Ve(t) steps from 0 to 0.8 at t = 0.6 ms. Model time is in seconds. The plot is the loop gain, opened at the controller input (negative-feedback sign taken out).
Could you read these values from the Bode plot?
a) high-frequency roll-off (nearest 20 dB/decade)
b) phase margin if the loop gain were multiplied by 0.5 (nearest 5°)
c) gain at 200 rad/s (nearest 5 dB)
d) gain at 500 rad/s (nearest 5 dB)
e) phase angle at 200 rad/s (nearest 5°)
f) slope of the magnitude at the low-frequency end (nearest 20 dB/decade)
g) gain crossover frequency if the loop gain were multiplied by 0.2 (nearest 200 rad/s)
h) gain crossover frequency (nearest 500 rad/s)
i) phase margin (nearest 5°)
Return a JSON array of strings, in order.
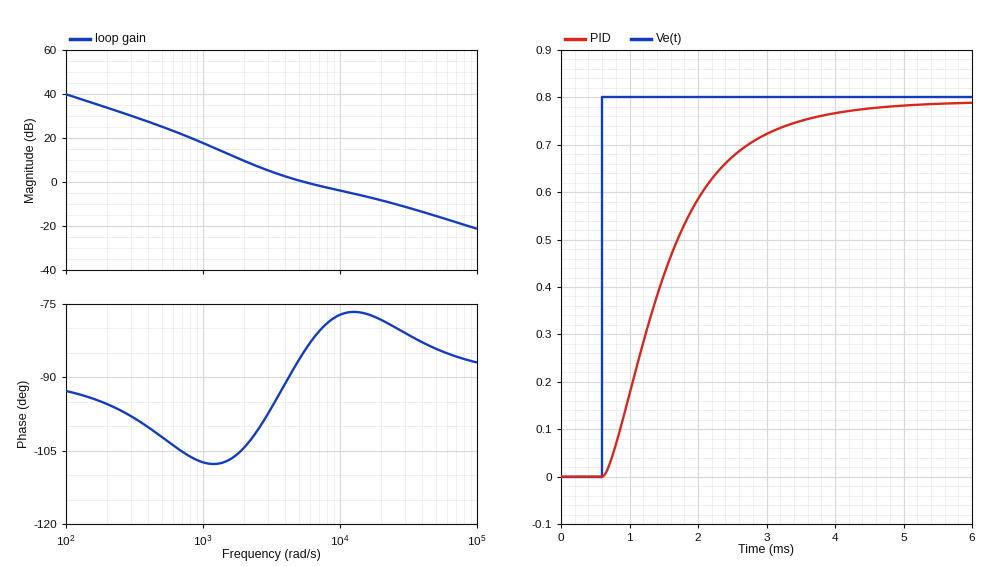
["-20 dB/decade", "80°", "35 dB", "25 dB", "-95°", "-20 dB/decade", "1400 rad/s", "5500 rad/s", "95°"]
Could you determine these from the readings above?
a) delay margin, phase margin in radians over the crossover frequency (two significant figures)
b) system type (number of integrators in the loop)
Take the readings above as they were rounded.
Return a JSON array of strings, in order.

["0.00030 s", "1"]
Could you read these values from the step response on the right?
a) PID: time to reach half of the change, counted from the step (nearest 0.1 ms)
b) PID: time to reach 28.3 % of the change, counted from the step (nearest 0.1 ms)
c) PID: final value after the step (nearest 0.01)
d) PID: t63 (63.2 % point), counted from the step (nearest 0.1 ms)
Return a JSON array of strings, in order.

["0.8 ms", "0.5 ms", "0.79", "1.1 ms"]
